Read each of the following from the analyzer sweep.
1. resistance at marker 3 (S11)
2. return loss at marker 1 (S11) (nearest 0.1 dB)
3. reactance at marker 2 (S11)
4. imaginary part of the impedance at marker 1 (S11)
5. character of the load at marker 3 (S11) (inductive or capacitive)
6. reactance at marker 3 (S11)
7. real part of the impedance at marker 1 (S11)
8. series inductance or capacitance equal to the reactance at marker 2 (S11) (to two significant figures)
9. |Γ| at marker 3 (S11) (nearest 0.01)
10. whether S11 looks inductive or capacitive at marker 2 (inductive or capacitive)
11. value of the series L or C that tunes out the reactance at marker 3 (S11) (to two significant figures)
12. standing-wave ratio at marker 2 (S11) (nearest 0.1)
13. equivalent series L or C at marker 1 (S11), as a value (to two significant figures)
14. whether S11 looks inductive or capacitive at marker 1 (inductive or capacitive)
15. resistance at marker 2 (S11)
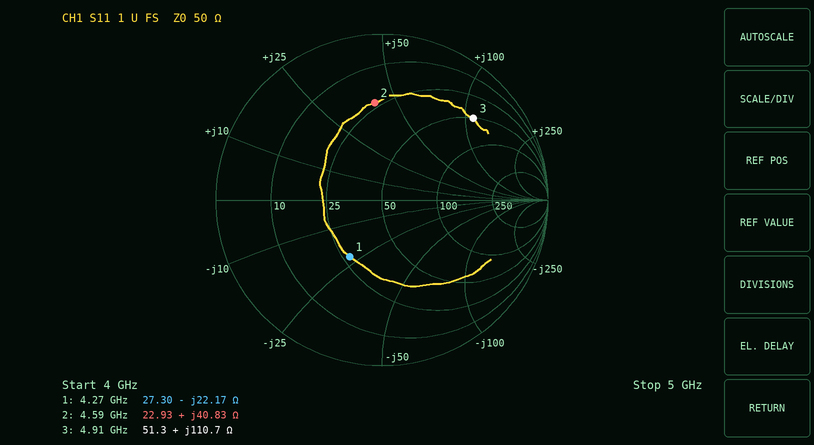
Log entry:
51.3 Ω
8.1 dB
+40.83 Ω
-22.17 Ω
inductive
+110.7 Ω
27.30 Ω
1.4 nH
0.74
inductive
290 fF
3.8
1.7 pF
capacitive
22.93 Ω
